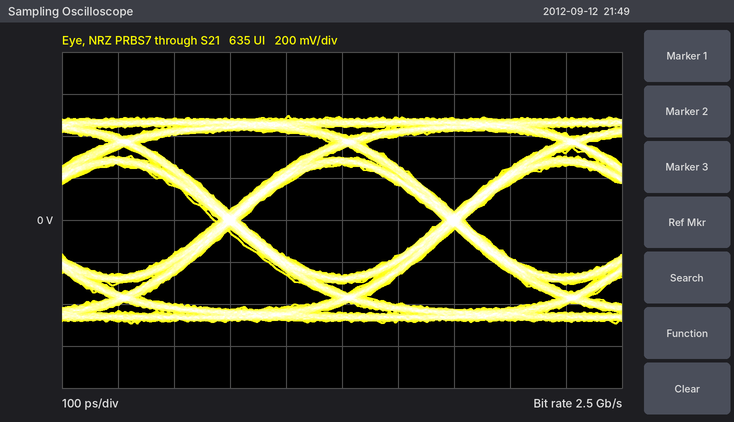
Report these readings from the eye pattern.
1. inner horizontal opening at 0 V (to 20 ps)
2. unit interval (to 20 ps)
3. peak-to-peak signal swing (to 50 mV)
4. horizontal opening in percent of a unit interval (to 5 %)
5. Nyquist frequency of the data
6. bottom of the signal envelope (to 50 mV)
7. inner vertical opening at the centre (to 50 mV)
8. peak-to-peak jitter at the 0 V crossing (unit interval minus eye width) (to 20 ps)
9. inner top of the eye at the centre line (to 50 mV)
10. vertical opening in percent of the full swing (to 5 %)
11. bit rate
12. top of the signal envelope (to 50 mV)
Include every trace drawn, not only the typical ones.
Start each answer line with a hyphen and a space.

- 360 ps
- 400 ps
- 1.00 V
- 90 %
- 1.25 GHz
- -500 mV
- 550 mV
- 40 ps
- 250 mV
- 55 %
- 2.5 Gb/s
- 500 mV
